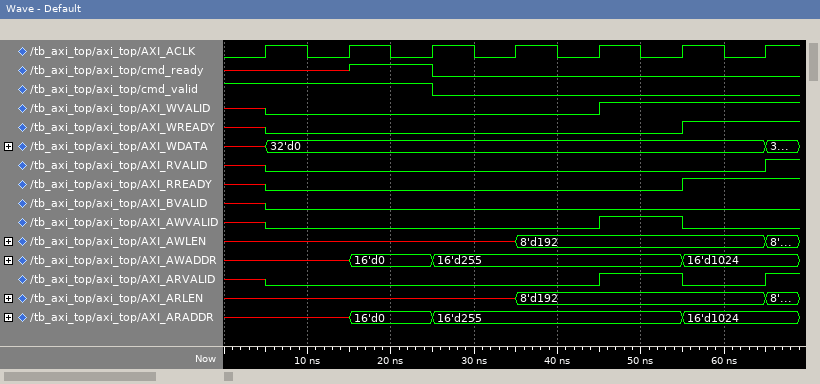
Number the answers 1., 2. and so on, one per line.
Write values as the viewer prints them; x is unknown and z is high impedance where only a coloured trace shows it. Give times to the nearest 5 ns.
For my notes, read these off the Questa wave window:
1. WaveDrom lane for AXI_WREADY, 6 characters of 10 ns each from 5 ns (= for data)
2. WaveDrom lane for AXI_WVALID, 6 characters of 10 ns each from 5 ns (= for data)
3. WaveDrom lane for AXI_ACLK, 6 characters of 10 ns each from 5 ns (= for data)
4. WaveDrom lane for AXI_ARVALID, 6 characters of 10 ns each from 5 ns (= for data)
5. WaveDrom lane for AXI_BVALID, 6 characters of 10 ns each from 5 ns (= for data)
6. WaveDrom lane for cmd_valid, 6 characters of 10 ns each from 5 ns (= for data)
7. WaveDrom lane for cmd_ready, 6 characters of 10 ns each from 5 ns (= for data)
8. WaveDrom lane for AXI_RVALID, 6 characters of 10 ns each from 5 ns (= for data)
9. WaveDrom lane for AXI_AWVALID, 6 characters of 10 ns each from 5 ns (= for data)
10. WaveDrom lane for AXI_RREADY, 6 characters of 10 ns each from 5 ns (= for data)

1. {name: 'AXI_WREADY', wave: '0....1'}
2. {name: 'AXI_WVALID', wave: '0...1.'}
3. {name: 'AXI_ACLK', wave: 'p.....'}
4. {name: 'AXI_ARVALID', wave: '0...10'}
5. {name: 'AXI_BVALID', wave: '0.....'}
6. {name: 'cmd_valid', wave: '1.0...'}
7. {name: 'cmd_ready', wave: 'x10...'}
8. {name: 'AXI_RVALID', wave: '0.....'}
9. {name: 'AXI_AWVALID', wave: '0...10'}
10. {name: 'AXI_RREADY', wave: '0....1'}
